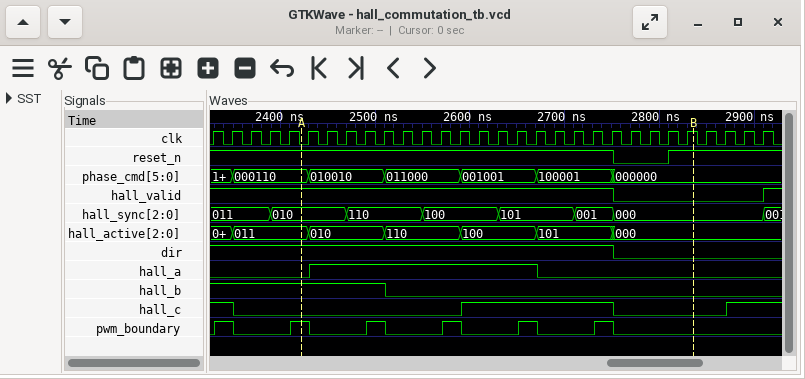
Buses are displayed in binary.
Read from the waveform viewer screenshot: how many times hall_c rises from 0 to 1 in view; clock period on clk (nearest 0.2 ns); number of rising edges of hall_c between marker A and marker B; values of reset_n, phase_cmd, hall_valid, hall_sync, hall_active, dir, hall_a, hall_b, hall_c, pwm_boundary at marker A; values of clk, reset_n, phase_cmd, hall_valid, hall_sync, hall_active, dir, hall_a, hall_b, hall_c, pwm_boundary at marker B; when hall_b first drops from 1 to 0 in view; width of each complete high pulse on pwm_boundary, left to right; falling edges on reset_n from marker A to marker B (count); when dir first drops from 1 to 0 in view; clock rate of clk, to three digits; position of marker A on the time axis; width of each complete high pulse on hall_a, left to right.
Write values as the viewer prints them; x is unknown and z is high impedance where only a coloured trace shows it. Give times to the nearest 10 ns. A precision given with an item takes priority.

2
20 ns
1
reset_n=1, phase_cmd=000110, hall_valid=1, hall_sync=010, hall_active=011, dir=1, hall_a=0, hall_b=1, hall_c=0, pwm_boundary=1
clk=1, reset_n=1, phase_cmd=000000, hall_valid=0, hall_sync=000, hall_active=000, dir=0, hall_a=0, hall_b=0, hall_c=0, pwm_boundary=0
2510 ns
20 ns, 20 ns, 20 ns, 20 ns, 20 ns, 20 ns
1
2750 ns
50.0 MHz
2420 ns
240 ns
